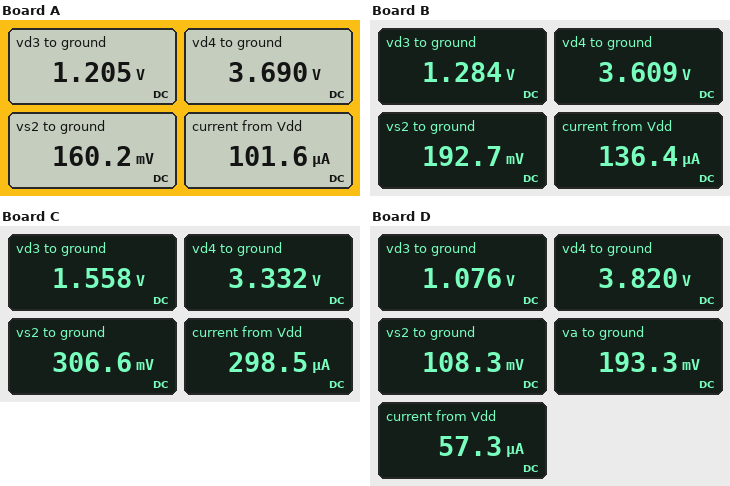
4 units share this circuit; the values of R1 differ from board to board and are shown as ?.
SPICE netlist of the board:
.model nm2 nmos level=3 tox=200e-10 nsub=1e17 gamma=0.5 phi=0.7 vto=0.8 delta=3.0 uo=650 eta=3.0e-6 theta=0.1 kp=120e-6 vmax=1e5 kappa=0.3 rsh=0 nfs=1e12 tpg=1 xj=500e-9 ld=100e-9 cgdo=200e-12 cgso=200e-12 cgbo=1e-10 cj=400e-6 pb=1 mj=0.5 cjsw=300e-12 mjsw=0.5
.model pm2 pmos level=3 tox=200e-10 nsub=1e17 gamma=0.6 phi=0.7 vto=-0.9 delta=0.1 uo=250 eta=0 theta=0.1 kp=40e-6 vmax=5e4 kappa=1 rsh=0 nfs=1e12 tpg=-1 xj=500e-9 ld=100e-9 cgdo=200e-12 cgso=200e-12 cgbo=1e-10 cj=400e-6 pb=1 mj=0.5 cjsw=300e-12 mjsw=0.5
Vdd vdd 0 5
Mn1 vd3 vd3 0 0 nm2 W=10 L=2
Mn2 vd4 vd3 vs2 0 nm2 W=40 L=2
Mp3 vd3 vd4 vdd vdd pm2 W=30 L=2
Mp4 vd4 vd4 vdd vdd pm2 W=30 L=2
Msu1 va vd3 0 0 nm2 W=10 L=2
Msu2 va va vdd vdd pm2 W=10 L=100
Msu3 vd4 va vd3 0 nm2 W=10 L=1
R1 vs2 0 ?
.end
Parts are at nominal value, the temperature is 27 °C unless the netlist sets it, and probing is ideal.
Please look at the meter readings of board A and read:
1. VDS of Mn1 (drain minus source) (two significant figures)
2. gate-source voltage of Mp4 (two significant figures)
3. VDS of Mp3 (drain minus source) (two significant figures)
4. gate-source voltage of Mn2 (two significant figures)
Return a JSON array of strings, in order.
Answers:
["1.2 V", "-1.3 V", "-3.8 V", "1.0 V"]
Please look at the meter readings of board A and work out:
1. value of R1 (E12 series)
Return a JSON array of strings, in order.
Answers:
["3.9 kΩ"]
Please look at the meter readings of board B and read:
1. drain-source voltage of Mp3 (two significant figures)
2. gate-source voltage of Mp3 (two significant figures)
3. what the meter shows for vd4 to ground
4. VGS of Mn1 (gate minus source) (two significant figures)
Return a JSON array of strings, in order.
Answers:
["-3.7 V", "-1.4 V", "3.609 V", "1.3 V"]
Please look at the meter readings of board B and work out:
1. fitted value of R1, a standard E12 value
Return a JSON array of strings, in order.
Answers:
["3.3 kΩ"]
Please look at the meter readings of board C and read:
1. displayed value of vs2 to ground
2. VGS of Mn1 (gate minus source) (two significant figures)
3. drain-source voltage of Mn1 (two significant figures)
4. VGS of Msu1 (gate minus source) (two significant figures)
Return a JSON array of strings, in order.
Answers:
["306.6 mV", "1.6 V", "1.6 V", "1.6 V"]
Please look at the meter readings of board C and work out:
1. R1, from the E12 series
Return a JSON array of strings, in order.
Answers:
["2.2 kΩ"]
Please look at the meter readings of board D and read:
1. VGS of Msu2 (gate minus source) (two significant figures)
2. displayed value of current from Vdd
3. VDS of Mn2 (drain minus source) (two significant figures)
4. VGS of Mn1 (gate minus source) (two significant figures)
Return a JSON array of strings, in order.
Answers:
["-4.8 V", "57.3 µA", "3.7 V", "1.1 V"]
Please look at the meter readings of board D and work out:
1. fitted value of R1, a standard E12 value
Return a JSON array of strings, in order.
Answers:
["5.6 kΩ"]
